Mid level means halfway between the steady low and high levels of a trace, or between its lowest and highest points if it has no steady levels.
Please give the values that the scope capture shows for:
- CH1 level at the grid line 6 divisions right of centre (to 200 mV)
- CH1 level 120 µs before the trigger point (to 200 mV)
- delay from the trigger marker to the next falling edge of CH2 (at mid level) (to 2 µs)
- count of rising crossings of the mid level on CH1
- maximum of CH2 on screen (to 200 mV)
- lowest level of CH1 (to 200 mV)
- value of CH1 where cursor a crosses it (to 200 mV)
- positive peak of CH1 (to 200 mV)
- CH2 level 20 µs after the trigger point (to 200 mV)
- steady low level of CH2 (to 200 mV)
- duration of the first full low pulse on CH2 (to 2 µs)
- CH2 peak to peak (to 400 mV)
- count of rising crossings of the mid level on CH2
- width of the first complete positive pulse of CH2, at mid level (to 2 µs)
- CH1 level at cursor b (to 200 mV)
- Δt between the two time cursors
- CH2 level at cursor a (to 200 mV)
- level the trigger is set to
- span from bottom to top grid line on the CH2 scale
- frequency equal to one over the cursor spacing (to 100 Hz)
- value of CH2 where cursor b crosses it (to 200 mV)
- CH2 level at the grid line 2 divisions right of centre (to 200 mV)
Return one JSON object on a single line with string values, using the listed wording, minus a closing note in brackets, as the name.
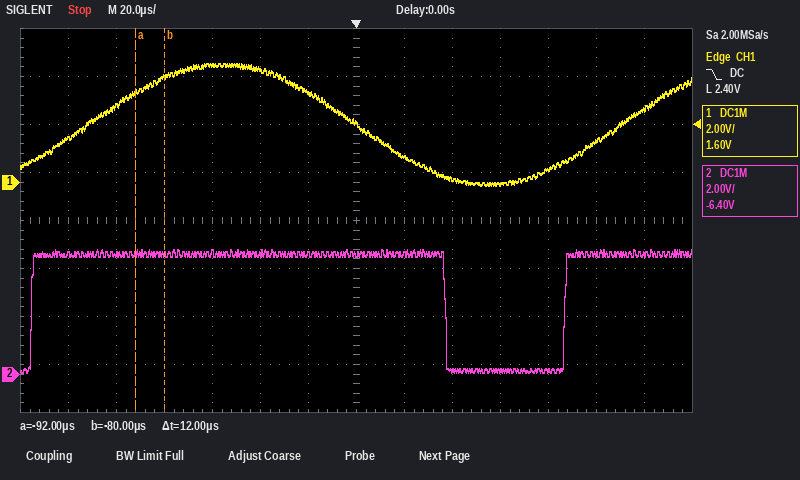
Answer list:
{"CH1 level at the grid line 6 divisions right of centre": "3.0 V", "CH1 level 120 µs before the trigger point": "1.8 V", "delay from the trigger marker to the next falling edge of CH2 (at mid level)": "38 µs", "count of rising crossings of the mid level on CH1": "2", "maximum of CH2 on screen": "5.2 V", "lowest level of CH1": "-200 mV", "value of CH1 where cursor a crosses it": "3.8 V", "positive peak of CH1": "5.0 V", "CH2 level 20 µs after the trigger point": "5.0 V", "steady low level of CH2": "200 mV", "duration of the first full low pulse on CH2": "50 µs", "CH2 peak to peak": "5.2 V", "count of rising crossings of the mid level on CH2": "2", "width of the first complete positive pulse of CH2, at mid level": "172 µs", "CH1 level at cursor b": "4.4 V", "Δt between the two time cursors": "12 µs", "CH2 level at cursor a": "5.0 V", "level the trigger is set to": "2.40 V", "span from bottom to top grid line on the CH2 scale": "16 V", "frequency equal to one over the cursor spacing": "83.3 kHz", "value of CH2 where cursor b crosses it": "5.0 V", "CH2 level at the grid line 2 divisions right of centre": "200 mV"}
